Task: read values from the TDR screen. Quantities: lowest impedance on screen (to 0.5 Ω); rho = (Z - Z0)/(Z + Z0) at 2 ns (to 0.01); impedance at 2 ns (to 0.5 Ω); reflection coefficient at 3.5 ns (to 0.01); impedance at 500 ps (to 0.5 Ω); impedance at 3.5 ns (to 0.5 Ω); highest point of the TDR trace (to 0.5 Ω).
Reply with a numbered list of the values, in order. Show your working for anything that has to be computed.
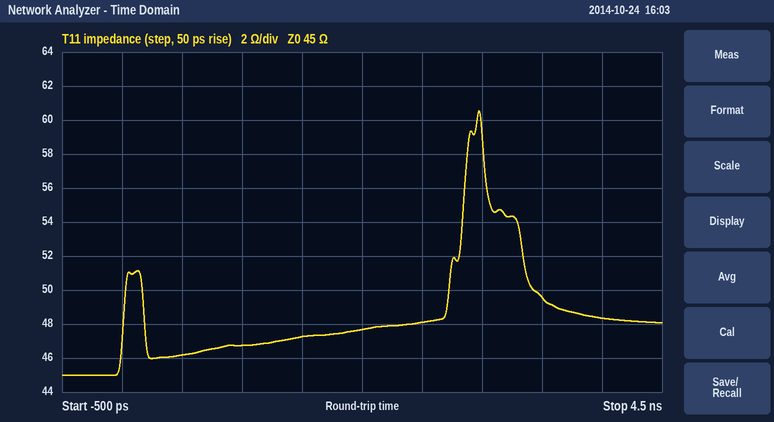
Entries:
1. 45.0 Ω
2. (47.5 − 45)/(47.5 + 45) ≈ +0.03
3. 47.5 Ω
4. (49.5 − 45)/(49.5 + 45) ≈ +0.05
5. 46.0 Ω
6. 49.5 Ω
7. 60.5 Ω
